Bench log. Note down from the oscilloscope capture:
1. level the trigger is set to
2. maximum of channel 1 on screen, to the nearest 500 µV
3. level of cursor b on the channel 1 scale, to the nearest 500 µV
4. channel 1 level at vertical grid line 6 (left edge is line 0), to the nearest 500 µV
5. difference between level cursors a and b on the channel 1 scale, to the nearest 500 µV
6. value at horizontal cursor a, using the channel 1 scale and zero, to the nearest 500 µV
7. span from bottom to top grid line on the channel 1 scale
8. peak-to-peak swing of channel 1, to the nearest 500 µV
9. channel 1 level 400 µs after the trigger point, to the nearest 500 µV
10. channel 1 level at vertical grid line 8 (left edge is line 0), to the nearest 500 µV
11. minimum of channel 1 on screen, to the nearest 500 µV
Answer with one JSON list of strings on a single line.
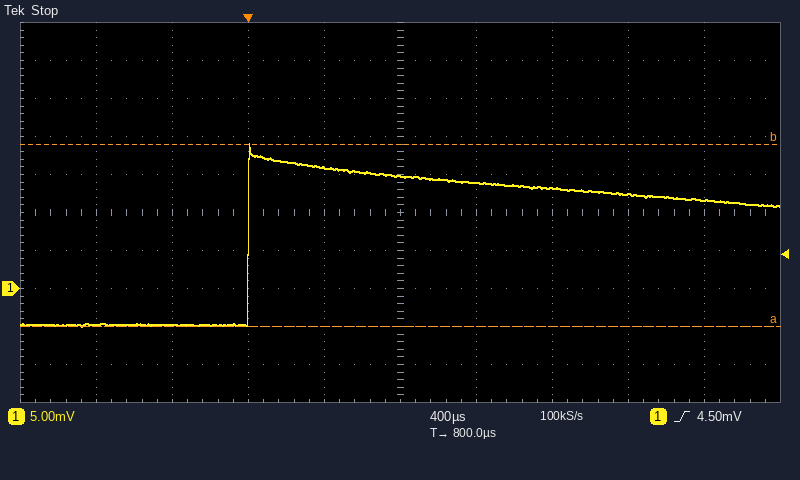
["4.50 mV", "19.0 mV", "19.0 mV", "14.0 mV", "24.0 mV", "-5.0 mV", "50 mV", "24.0 mV", "16.0 mV", "12.5 mV", "-5.0 mV"]
